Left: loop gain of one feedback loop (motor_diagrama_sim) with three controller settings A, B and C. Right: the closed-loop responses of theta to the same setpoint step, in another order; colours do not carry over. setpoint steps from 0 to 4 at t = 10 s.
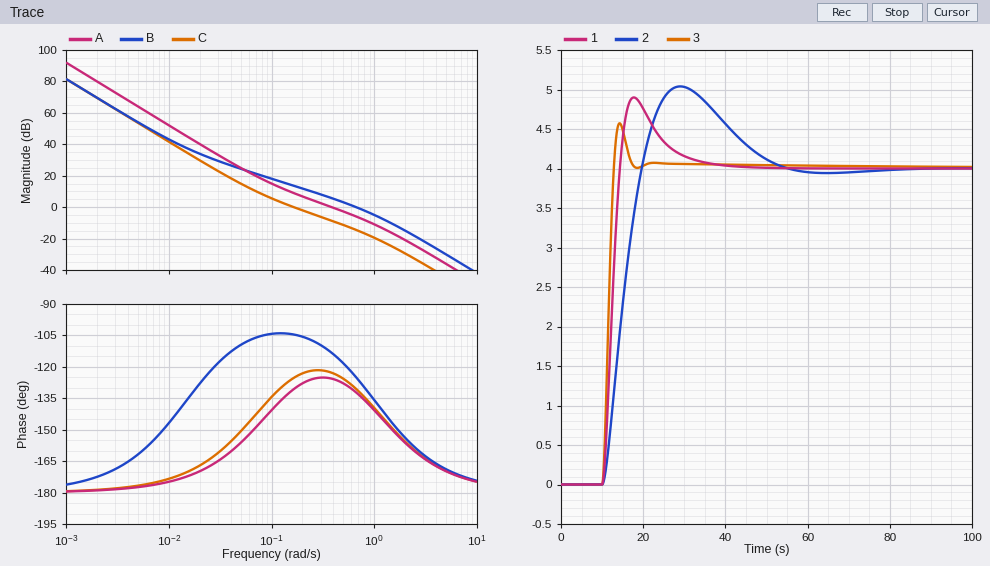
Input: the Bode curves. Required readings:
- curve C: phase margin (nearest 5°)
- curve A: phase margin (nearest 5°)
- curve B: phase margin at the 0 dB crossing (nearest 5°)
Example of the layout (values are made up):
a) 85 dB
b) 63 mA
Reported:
a) 55°
b) 55°
c) 55°
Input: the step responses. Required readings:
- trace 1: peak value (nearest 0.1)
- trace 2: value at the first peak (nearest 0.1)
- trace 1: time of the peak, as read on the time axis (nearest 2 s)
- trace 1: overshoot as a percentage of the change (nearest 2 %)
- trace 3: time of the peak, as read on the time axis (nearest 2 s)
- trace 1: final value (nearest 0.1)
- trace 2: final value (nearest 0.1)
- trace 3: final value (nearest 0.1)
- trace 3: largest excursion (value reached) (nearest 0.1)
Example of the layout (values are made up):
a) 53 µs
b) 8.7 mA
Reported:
a) 4.9
b) 5.0
c) 18 s
d) 22 %
e) 14 s
f) 4.0
g) 4.0
h) 4.0
i) 4.6
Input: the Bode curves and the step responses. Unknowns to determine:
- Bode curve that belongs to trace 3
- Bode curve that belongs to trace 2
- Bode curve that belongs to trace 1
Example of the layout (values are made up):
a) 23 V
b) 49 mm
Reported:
a) B
b) C
c) A
